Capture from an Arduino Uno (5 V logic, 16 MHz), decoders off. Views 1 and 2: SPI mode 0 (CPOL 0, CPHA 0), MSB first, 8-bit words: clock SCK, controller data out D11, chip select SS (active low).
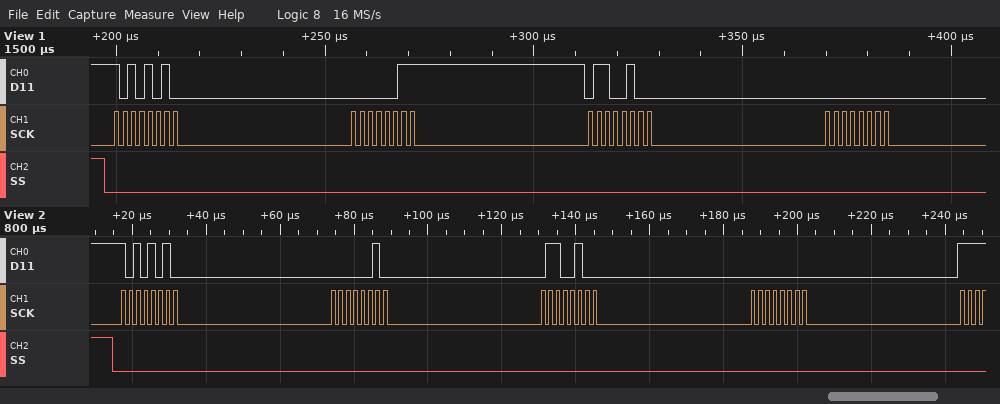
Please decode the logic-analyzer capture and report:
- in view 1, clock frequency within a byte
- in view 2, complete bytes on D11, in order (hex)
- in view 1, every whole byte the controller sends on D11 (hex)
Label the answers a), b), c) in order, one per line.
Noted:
a) 500 kHz
b) 0xAA 0x02 0x64 0x00
c) 0xAA 0x03 0x64 0x00
